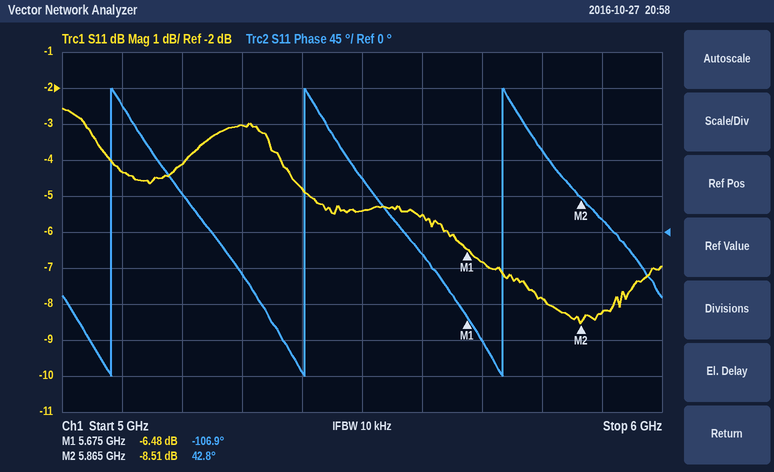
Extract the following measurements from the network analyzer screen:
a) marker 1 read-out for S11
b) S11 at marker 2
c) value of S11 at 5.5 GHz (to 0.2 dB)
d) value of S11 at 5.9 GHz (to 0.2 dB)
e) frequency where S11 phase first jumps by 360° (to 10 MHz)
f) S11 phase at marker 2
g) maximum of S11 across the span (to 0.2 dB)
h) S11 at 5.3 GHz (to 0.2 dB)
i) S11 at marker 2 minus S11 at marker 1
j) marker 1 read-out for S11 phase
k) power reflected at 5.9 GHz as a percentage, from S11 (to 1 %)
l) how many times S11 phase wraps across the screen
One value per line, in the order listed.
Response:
-6.48 dB
-8.51 dB
-5.4 dB
-8.2 dB
5.08 GHz
42.8°
-2.6 dB
-3.0 dB
-2.03 dB
-106.9°
15 %
3
